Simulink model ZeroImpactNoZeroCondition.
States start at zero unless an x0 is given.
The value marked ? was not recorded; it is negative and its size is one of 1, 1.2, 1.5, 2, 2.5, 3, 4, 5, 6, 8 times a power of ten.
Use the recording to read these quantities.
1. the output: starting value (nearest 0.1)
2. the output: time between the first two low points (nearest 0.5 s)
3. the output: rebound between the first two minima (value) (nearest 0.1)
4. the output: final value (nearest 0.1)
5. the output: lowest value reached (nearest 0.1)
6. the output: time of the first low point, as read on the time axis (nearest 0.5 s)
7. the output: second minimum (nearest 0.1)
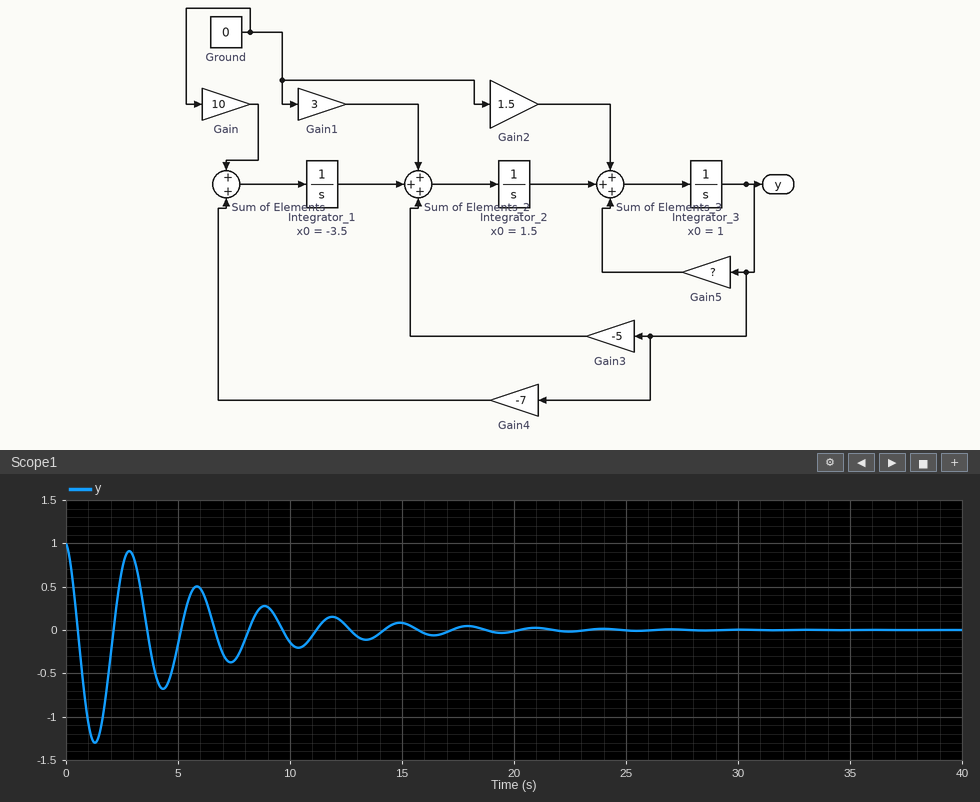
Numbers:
1.0
3.0 s
0.9
0.0
-1.3
1.5 s
-0.7
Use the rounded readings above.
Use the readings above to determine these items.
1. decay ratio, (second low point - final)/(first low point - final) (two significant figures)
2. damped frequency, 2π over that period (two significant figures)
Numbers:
0.54
2.1 rad/s
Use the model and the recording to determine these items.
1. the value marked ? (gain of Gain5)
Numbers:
-2
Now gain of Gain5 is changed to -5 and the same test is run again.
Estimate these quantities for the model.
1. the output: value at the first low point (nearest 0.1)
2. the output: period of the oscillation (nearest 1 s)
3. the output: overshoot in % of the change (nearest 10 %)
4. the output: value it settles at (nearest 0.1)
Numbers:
-0.6
5 s
60 %
0.0
